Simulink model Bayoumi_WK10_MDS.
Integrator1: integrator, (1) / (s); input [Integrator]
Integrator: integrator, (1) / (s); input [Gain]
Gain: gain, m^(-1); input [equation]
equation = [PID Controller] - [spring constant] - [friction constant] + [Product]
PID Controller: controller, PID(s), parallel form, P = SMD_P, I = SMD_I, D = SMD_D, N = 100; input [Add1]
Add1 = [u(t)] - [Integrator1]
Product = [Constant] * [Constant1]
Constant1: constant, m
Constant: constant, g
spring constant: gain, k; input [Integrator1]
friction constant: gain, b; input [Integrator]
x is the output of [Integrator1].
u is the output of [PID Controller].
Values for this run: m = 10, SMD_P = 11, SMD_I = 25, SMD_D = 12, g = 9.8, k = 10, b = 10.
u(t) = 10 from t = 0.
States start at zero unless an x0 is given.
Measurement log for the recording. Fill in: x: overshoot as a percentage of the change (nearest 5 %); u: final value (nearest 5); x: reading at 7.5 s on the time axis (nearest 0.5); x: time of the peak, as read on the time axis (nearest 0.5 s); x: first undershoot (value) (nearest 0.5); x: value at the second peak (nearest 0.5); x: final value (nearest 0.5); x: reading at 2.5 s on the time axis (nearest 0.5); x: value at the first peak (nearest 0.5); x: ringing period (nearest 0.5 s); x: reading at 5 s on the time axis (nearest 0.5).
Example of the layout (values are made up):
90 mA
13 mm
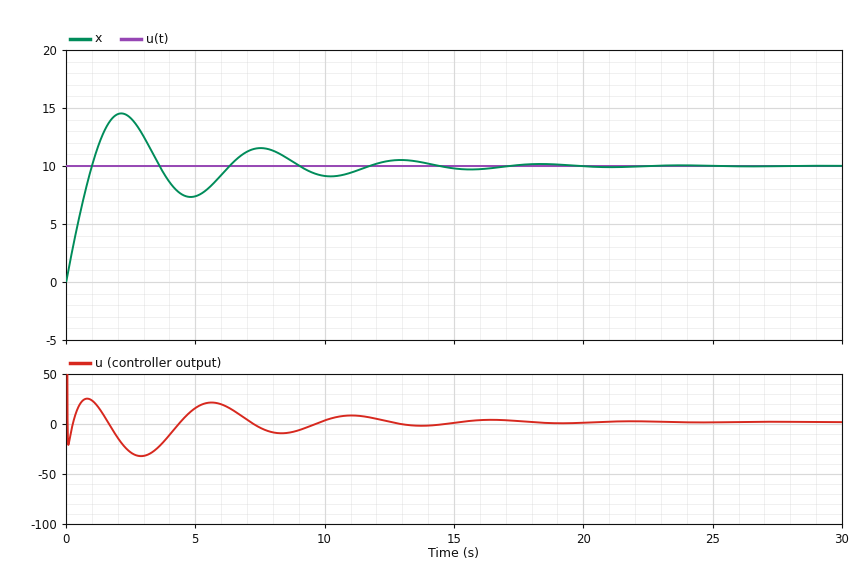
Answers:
45 %
0
11.5
2.0 s
7.5
11.5
10.0
14.0
14.5
5.5 s
7.5
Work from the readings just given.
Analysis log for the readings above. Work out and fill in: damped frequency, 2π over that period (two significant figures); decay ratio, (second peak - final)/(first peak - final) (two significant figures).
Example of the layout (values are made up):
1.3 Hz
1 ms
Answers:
1.1 rad/s
0.33
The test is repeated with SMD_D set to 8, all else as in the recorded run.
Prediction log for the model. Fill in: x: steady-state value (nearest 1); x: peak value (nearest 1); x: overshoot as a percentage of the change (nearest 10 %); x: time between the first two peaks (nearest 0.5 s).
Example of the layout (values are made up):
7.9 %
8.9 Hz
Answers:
10
16
60 %
5.0 s
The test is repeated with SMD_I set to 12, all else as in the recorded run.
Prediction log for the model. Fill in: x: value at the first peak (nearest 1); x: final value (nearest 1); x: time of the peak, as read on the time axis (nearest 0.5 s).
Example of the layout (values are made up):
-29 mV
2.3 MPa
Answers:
13
10
2.5 s
